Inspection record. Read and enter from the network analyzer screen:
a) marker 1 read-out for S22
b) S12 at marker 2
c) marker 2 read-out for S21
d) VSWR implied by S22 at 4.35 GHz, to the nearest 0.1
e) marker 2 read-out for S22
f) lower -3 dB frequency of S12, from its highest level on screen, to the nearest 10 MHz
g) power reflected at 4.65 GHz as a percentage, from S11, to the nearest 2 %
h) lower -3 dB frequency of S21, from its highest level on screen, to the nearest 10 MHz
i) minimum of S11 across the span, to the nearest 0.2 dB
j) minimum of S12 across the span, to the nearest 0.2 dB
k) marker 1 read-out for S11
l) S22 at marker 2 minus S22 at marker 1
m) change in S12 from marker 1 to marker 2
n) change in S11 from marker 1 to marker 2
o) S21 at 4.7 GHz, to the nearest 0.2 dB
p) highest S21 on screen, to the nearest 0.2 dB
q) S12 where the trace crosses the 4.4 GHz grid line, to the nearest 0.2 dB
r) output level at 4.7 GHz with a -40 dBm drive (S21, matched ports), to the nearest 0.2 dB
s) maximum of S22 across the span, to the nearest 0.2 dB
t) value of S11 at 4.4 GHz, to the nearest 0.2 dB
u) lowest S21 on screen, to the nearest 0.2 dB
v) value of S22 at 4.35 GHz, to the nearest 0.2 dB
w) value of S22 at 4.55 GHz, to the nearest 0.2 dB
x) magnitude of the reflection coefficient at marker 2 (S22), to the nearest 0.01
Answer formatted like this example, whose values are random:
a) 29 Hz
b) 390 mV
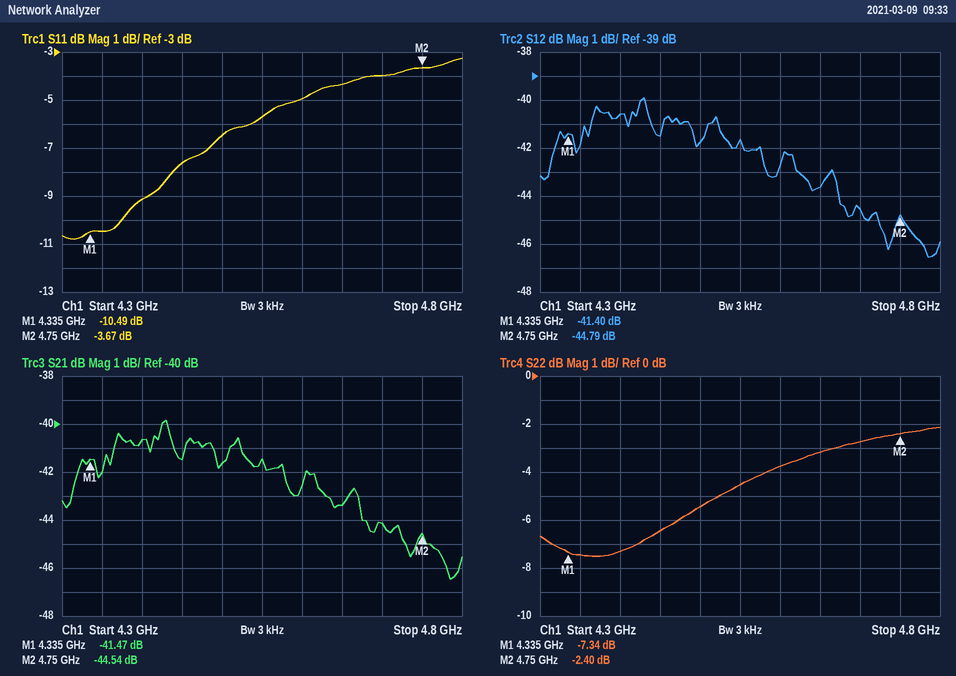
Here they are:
a) -7.34 dB
b) -44.79 dB
c) -44.54 dB
d) 2.5
e) -2.40 dB
f) 4.31 GHz
g) 36 %
h) 4.31 GHz
i) -10.8 dB
j) -46.6 dB
k) -10.49 dB
l) 4.94 dB
m) -3.39 dB
n) 6.82 dB
o) -44.2 dB
p) -39.8 dB
q) -40.6 dB
r) -84.2 dBm
s) -2.2 dB
t) -9.2 dB
u) -46.4 dB
v) -7.4 dB
w) -4.6 dB
x) 0.76
